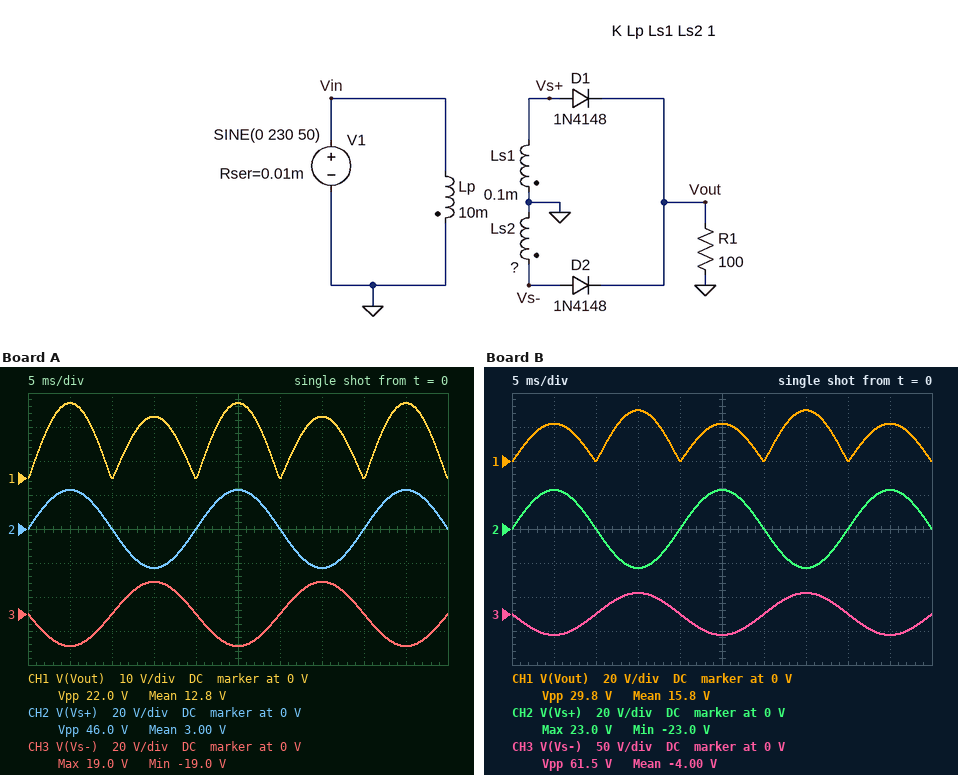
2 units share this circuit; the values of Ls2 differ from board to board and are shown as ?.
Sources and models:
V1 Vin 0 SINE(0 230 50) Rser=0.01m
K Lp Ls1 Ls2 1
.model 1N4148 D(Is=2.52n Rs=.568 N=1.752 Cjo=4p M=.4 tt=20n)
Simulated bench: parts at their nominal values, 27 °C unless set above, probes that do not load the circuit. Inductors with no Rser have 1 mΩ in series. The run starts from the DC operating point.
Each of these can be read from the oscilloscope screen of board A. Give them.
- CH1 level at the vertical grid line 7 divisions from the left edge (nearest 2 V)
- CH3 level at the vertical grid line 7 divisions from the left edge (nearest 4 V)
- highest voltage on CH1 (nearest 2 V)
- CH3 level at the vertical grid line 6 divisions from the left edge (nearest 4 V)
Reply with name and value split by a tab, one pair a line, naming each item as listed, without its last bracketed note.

CH1 level at the vertical grid line 7 divisions from the left edge	18 V
CH3 level at the vertical grid line 7 divisions from the left edge	20 V
highest voltage on CH1	22 V
CH3 level at the vertical grid line 6 divisions from the left edge	0 V
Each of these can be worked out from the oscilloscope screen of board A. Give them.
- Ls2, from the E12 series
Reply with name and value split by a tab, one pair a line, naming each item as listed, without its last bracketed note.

Ls2, from the E12 series	68 µH
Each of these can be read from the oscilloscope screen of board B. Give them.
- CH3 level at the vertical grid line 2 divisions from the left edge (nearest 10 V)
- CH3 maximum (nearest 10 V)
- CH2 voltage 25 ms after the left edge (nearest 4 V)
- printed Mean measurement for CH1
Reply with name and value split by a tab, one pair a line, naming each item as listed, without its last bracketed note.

CH3 level at the vertical grid line 2 divisions from the left edge	0 V
CH3 maximum	30 V
CH2 voltage 25 ms after the left edge	24 V
printed Mean measurement for CH1	15.8 V
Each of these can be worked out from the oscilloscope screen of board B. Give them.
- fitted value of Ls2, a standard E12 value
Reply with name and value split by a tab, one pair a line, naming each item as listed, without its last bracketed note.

fitted value of Ls2, a standard E12 value	180 µH
